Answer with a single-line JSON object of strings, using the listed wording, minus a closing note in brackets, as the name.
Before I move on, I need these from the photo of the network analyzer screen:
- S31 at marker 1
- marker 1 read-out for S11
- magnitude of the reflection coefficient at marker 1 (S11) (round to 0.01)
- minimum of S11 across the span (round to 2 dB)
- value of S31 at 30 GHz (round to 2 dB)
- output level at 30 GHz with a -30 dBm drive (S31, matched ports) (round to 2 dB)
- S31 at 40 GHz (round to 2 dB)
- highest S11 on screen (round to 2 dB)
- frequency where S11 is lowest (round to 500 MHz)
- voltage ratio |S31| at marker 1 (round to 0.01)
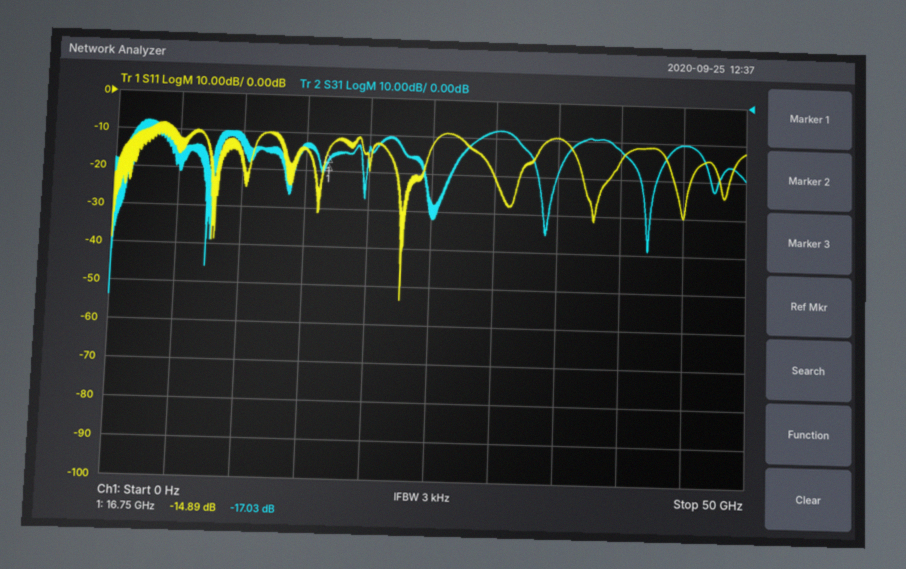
{"S31 at marker 1": "-17.03 dB", "marker 1 read-out for S11": "-14.89 dB", "magnitude of the reflection coefficient at marker 1 (S11)": "0.18", "minimum of S11 across the span": "-54 dB", "value of S31 at 30 GHz": "-8 dB", "output level at 30 GHz with a -30 dBm drive (S31, matched ports)": "-38 dBm", "S31 at 40 GHz": "-12 dB", "highest S11 on screen": "-8 dB", "frequency where S11 is lowest": "22.5 GHz", "voltage ratio |S31| at marker 1": "0.14"}
